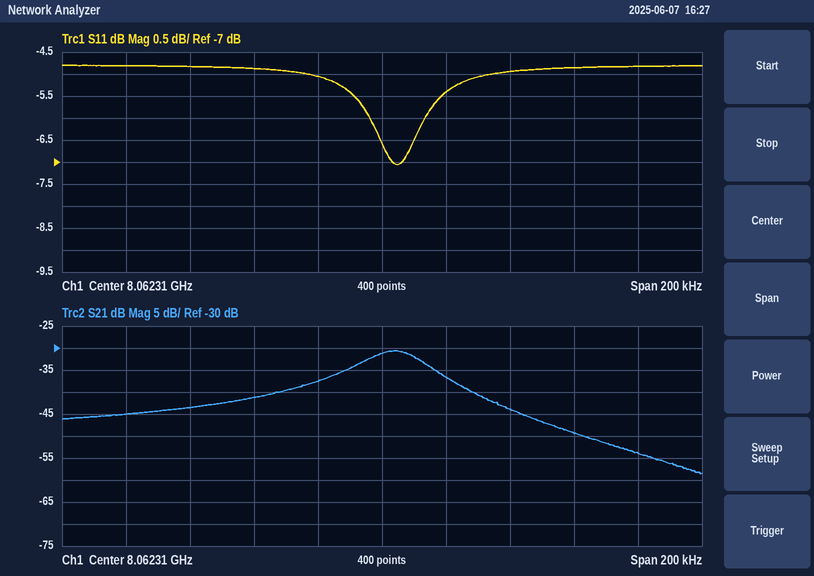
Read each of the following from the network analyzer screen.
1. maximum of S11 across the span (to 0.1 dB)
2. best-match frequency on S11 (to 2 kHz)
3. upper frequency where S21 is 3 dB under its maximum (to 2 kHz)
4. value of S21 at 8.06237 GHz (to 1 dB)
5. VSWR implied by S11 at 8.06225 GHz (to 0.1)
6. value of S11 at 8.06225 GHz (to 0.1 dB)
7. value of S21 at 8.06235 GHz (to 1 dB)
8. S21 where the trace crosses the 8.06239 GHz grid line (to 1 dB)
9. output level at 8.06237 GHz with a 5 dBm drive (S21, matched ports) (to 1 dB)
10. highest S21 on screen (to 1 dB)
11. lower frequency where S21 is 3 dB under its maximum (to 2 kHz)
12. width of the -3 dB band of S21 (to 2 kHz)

-4.8 dB
8.062314 GHz
8.062324 GHz
-49 dB
3.7
-4.8 dB
-44 dB
-54 dB
-44 dBm
-31 dB
8.062302 GHz
22 kHz
